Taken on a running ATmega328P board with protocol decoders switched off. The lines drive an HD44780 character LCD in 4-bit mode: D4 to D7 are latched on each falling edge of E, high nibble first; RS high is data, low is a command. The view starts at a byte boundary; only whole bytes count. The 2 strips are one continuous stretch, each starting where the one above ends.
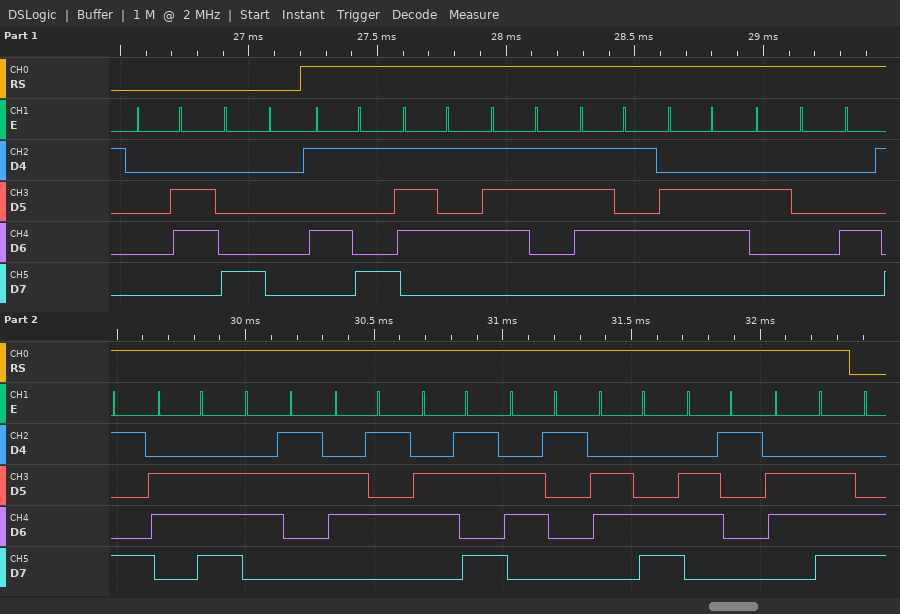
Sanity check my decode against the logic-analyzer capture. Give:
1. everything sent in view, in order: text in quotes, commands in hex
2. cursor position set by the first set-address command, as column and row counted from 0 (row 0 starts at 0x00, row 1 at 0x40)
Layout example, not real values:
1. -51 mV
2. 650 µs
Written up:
1. 0x06 0x80 "Yusuf Incekalan"
2. column 0, row 0
